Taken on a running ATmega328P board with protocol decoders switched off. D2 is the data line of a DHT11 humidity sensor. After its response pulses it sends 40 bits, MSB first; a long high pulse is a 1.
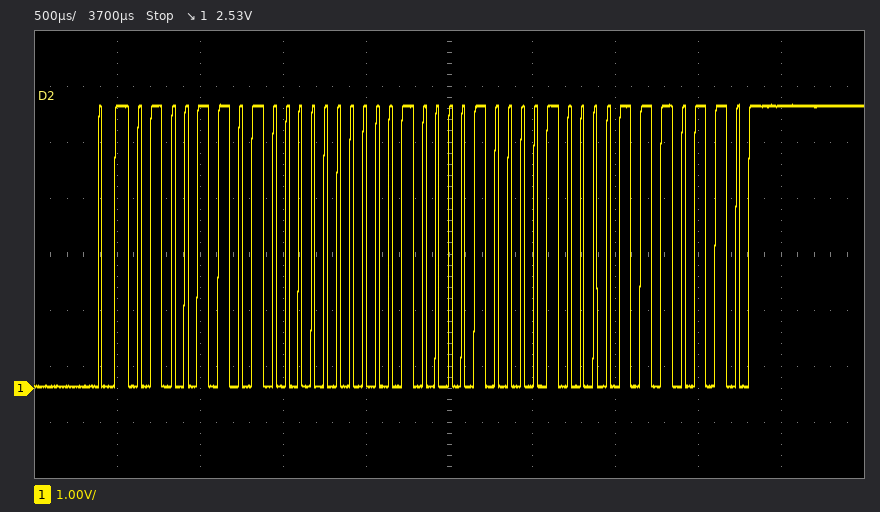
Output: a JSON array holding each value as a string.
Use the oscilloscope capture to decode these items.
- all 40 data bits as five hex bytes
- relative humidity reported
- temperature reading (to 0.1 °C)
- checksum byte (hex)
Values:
["4D 00 21 08 76", "77 %", "33.8 °C", "0x76"]
